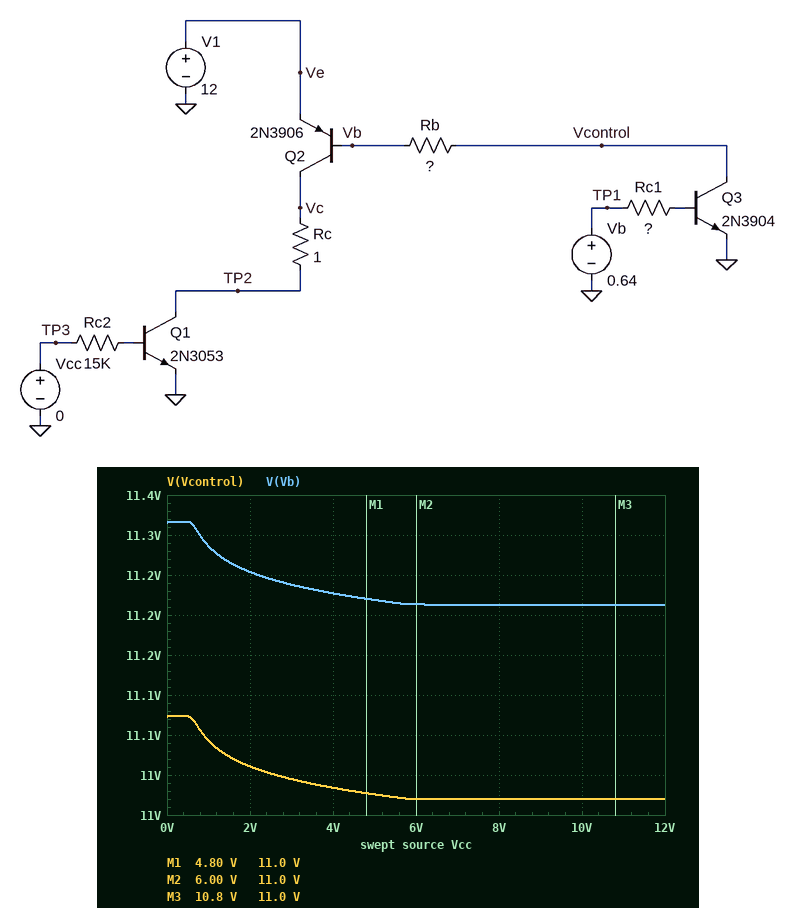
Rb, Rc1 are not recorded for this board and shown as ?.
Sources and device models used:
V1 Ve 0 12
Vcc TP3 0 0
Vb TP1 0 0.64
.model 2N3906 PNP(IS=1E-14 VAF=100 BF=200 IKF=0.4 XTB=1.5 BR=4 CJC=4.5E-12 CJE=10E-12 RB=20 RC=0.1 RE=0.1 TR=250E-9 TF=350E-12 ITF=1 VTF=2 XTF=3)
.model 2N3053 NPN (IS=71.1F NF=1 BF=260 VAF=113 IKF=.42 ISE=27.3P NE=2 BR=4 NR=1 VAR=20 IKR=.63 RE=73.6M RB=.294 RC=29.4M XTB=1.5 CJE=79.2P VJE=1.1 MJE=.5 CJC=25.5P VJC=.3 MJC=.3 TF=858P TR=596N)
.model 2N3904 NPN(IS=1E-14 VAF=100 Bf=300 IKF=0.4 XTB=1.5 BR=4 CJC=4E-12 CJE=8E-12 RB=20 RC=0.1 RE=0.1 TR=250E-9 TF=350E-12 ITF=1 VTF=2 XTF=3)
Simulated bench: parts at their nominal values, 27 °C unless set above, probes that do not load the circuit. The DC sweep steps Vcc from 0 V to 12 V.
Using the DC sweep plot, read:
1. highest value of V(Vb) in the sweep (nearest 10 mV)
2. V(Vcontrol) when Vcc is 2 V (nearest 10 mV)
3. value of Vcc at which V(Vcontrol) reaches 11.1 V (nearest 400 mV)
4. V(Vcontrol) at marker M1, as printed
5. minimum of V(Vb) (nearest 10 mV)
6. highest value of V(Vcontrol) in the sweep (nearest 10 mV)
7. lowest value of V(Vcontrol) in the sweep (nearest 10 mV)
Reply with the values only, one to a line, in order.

11.32 V
11.01 V
800 mV
11.0 V
11.21 V
11.07 V
10.97 V
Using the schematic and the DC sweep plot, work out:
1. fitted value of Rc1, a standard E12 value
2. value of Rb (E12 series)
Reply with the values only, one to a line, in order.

6.8 kΩ
560 Ω
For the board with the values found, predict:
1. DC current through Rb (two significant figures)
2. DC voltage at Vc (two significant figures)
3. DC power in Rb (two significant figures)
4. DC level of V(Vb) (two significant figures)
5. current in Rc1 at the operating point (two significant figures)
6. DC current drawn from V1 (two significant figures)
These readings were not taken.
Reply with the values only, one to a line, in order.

430 µA
12 V
110 µW
11 V
1.3 µA
430 µA
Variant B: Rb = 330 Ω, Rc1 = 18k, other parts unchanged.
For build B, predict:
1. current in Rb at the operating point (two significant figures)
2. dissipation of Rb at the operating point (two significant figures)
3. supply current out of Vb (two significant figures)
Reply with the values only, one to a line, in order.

320 µA
33 µW
950 nA
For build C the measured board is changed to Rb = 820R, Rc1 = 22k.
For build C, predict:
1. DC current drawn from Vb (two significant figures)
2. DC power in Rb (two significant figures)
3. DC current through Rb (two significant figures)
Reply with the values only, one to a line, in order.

880 nA
69 µW
290 µA
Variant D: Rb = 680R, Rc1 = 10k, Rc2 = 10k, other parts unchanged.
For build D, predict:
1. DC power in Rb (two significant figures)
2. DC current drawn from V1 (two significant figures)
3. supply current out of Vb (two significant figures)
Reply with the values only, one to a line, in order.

100 µW
390 µA
1.2 µA
